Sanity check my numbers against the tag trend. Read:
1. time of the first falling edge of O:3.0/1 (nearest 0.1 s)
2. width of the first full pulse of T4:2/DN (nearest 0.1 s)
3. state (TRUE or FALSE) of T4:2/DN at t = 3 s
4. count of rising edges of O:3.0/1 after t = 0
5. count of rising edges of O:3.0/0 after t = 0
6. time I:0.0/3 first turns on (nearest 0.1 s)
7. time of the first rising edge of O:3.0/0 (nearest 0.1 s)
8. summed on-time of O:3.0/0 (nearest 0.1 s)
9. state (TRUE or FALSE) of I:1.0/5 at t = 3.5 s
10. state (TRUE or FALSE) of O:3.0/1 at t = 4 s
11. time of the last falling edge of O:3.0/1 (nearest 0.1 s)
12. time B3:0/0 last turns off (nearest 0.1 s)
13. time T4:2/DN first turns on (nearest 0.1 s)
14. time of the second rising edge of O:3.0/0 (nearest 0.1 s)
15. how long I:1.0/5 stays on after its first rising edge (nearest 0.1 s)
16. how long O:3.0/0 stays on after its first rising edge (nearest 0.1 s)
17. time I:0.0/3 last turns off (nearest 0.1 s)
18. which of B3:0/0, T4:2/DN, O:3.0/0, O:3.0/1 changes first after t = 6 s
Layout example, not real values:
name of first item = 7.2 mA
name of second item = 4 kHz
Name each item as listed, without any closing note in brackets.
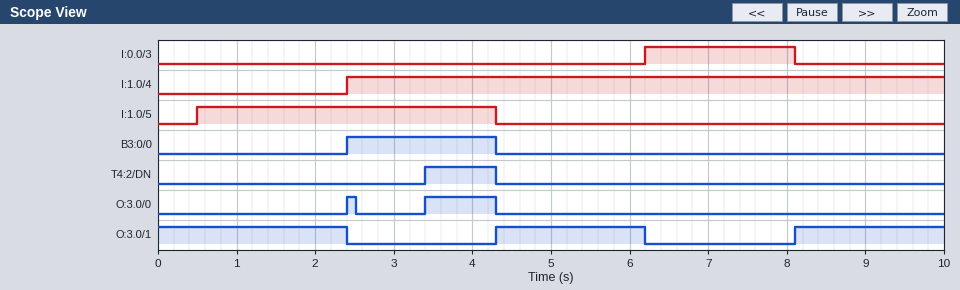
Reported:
time of the first falling edge of O:3.0/1 = 2.4 s
width of the first full pulse of T4:2/DN = 0.9 s
state (TRUE or FALSE) of T4:2/DN at t = 3 s = FALSE
count of rising edges of O:3.0/1 after t = 0 = 2
count of rising edges of O:3.0/0 after t = 0 = 2
time I:0.0/3 first turns on = 6.2 s
time of the first rising edge of O:3.0/0 = 2.4 s
summed on-time of O:3.0/0 = 1.0 s
state (TRUE or FALSE) of I:1.0/5 at t = 3.5 s = TRUE
state (TRUE or FALSE) of O:3.0/1 at t = 4 s = FALSE
time of the last falling edge of O:3.0/1 = 6.2 s
time B3:0/0 last turns off = 4.3 s
time T4:2/DN first turns on = 3.4 s
time of the second rising edge of O:3.0/0 = 3.4 s
how long I:1.0/5 stays on after its first rising edge = 3.8 s
how long O:3.0/0 stays on after its first rising edge = 0.1 s
time I:0.0/3 last turns off = 8.1 s
which of B3:0/0, T4:2/DN, O:3.0/0, O:3.0/1 changes first after t = 6 s = O:3.0/1
